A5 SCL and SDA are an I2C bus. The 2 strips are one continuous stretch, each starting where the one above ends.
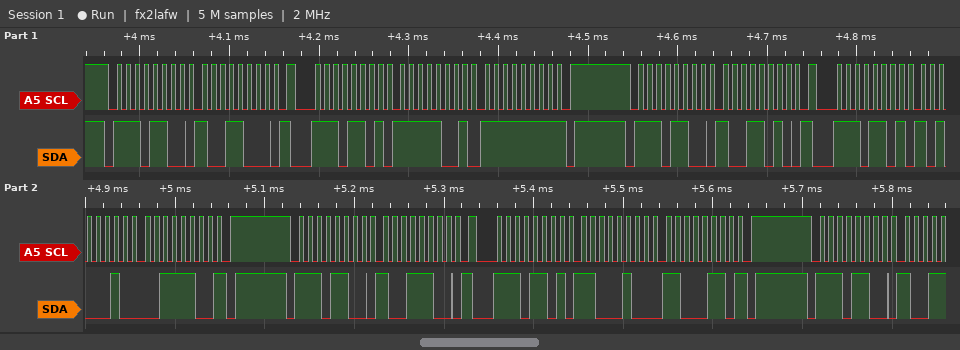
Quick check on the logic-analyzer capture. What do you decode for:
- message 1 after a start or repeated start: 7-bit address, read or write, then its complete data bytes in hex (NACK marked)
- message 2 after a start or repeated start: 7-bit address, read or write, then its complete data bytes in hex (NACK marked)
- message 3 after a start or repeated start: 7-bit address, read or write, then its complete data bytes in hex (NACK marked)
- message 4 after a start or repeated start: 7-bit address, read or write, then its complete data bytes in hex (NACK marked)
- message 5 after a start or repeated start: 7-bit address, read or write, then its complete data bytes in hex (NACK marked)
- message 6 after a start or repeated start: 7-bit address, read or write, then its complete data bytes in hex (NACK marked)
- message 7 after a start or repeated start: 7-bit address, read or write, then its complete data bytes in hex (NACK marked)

0x76 write: 98
0x76 read: F9 FF NACK
0x76 write: 9A
0x76 read: A2 3C NACK
0x76 write: 9C
0x76 read: C4 C6 NACK
0x76 write
